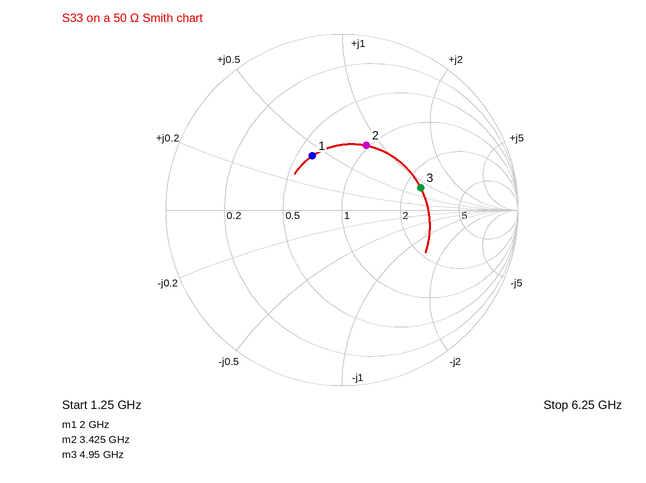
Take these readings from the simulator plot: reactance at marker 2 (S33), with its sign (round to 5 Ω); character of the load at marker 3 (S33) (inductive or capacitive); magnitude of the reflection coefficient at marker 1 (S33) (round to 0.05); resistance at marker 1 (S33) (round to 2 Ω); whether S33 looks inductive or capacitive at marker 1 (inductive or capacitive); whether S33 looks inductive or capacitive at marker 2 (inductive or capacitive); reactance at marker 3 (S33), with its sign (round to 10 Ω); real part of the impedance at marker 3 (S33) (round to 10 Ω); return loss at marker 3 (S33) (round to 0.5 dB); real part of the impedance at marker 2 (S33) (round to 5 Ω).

+40 Ω
inductive
0.35
30 Ω
inductive
inductive
+40 Ω
120 Ω
6.5 dB
50 Ω
